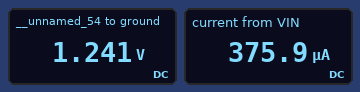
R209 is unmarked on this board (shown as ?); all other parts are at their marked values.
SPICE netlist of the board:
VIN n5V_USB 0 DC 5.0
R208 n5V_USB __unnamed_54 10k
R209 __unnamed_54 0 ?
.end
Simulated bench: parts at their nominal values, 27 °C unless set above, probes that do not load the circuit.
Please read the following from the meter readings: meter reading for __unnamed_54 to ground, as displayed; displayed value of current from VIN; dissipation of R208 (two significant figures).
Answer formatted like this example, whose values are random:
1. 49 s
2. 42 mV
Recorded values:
1. 1.241 V
2. 375.9 µA
3. 1.4 mW
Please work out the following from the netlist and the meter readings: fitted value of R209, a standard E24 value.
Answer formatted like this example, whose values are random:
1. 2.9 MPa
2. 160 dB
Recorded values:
1. 3.3 kΩ
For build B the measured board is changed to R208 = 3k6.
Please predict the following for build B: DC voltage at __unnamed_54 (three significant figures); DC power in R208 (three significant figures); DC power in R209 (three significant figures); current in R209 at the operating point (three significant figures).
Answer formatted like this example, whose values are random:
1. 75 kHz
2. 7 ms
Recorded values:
1. 2.39 V
2. 1.89 mW
3. 1.73 mW
4. 725 µA
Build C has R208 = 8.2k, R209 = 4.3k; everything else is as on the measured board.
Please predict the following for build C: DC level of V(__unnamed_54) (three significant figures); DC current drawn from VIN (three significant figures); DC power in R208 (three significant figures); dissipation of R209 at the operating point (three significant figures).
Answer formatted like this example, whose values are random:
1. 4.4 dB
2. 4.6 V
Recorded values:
1. 1.72 V
2. 400 µA
3. 1.31 mW
4. 688 µW
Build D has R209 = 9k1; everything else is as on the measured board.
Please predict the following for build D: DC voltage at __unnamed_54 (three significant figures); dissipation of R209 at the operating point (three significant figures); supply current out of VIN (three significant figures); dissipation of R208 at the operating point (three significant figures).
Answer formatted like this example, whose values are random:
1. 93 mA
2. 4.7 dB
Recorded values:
1. 2.38 V
2. 624 µW
3. 262 µA
4. 685 µW
